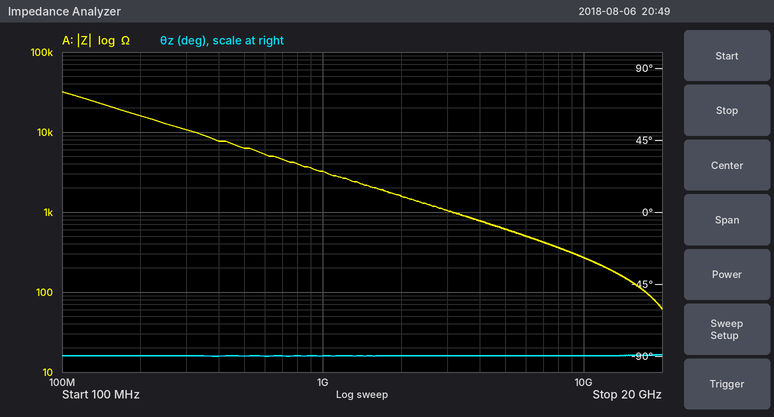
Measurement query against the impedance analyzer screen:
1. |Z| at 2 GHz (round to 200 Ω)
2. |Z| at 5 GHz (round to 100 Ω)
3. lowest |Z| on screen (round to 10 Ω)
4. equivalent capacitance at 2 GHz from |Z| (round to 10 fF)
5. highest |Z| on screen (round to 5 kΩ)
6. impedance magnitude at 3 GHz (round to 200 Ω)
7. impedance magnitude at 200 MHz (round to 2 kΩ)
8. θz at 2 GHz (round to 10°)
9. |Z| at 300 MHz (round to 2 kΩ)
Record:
1.6 kΩ
600 Ω
60 Ω
50 fF
30 kΩ
1.0 kΩ
16 kΩ
-90°
10 kΩ
